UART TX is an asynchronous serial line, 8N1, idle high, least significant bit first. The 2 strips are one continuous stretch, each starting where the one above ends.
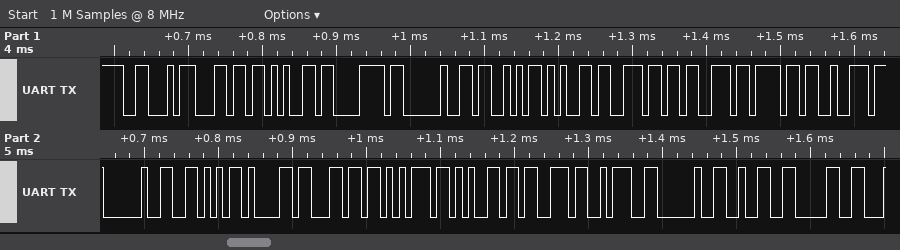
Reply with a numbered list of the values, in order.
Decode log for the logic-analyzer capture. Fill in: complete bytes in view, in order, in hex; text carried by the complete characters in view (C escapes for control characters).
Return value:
1. 46 6C 65 78 20 53 65 6E 73 6F 72 20 56 61 6C 75 65 73 3A 20 32 30
2. "Flex Sensor Values: 20"
